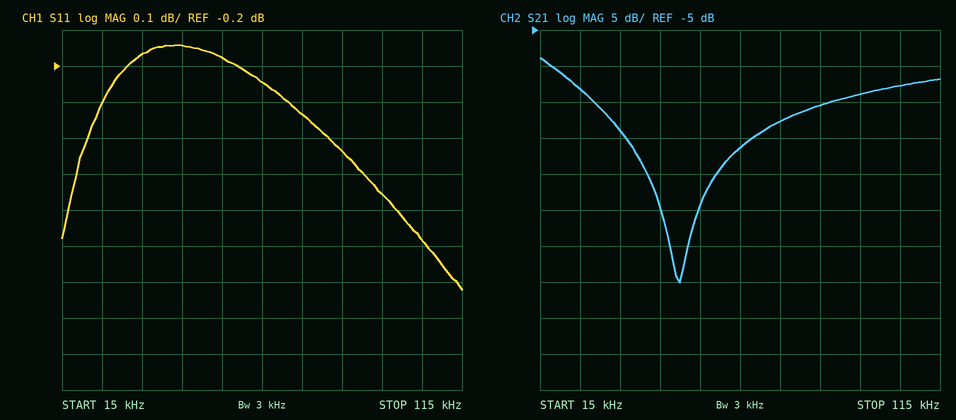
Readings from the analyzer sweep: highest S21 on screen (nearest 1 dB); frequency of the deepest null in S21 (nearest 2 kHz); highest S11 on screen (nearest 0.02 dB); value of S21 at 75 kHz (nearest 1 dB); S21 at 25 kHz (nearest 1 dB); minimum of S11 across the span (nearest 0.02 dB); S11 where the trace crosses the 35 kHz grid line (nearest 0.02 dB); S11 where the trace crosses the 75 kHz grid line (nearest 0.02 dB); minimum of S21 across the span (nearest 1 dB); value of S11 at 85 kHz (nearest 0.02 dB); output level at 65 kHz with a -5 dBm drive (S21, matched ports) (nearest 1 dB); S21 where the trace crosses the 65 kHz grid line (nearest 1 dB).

-9 dB
50 kHz
-0.14 dB
-18 dB
-13 dB
-0.82 dB
-0.16 dB
-0.34 dB
-40 dB
-0.44 dB
-26 dBm
-21 dB
